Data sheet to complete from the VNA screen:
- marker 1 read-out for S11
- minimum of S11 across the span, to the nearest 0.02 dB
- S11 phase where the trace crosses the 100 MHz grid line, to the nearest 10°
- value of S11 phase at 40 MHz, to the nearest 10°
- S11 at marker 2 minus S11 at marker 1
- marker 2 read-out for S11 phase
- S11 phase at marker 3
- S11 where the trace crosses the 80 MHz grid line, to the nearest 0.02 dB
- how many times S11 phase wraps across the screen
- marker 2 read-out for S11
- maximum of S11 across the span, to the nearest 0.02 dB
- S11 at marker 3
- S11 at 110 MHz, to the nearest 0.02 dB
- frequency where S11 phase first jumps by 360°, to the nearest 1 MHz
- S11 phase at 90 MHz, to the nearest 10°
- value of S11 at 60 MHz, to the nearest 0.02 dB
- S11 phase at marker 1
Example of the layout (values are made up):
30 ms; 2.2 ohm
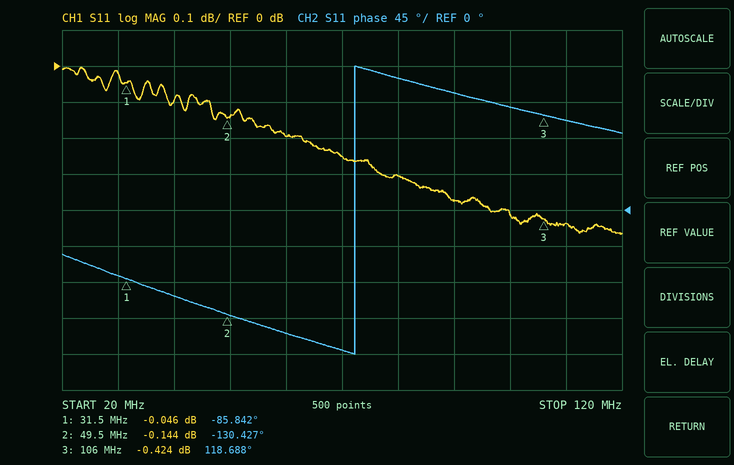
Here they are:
-0.046 dB; -0.46 dB; 130°; -110°; -0.098 dB; -130.427°; 118.688°; -0.30 dB; 1; -0.144 dB; 0.00 dB; -0.424 dB; -0.44 dB; 72 MHz; 150°; -0.20 dB; -85.842°
